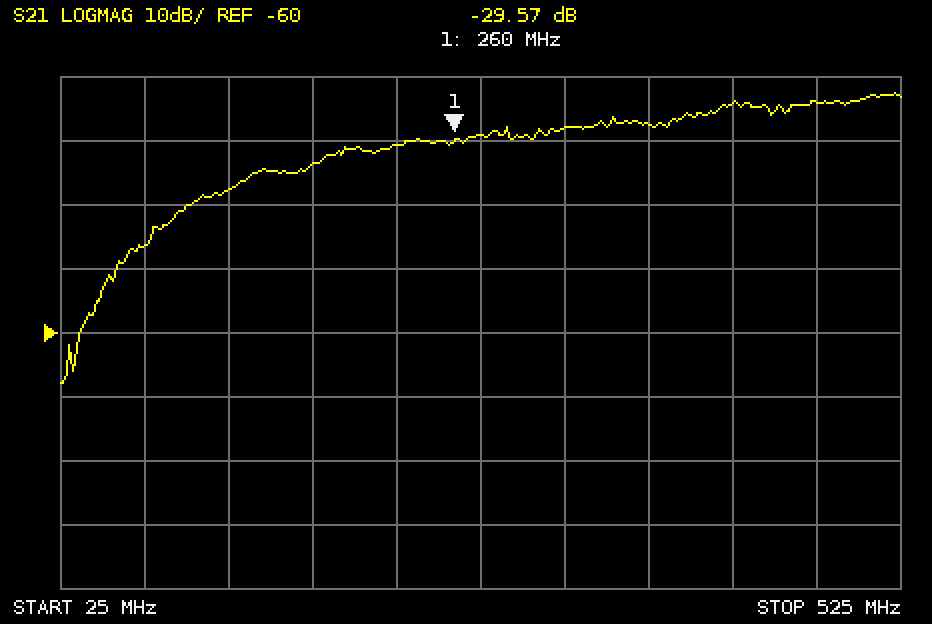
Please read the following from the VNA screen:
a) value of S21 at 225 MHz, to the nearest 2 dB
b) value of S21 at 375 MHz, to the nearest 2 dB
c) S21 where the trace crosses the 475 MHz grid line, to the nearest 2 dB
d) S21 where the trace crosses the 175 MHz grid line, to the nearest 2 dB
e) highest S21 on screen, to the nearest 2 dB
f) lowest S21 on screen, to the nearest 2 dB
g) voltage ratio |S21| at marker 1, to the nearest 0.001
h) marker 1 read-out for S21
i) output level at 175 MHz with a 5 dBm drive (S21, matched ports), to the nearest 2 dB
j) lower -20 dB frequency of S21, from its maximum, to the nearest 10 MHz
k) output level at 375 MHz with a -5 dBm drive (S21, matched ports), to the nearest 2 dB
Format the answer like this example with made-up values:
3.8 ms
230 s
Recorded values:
-30 dB
-28 dB
-24 dB
-34 dB
-22 dB
-68 dB
0.033
-29.57 dB
-28 dBm
90 MHz
-32 dBm
